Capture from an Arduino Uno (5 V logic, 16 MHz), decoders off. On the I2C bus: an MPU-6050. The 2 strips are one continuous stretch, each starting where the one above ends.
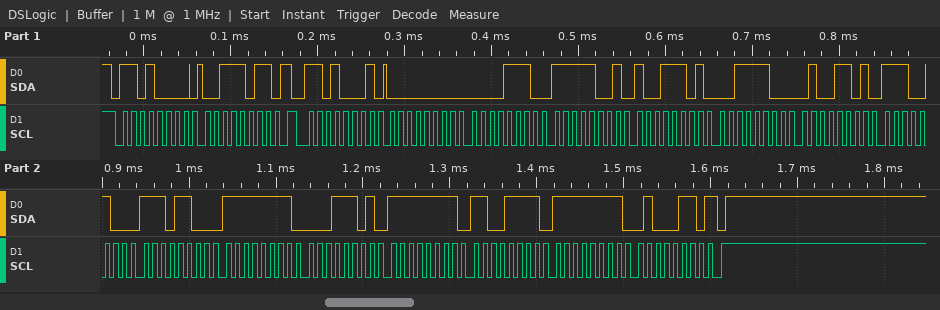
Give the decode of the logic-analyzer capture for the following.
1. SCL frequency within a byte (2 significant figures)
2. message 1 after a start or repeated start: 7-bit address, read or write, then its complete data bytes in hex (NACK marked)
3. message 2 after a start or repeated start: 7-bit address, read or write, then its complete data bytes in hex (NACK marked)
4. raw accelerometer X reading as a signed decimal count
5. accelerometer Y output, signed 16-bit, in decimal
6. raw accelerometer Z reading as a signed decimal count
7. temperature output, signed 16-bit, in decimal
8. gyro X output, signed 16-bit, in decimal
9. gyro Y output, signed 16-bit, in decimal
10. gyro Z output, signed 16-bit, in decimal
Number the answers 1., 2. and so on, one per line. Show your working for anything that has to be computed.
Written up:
1. 100 kHz
2. 0x68 write: 3B
3. 0x68 read: 00 0E F9 9D 3C 4D E4 EC FF 1D FF CF FF 46 NACK
4. 0x000E = 14
5. 0xF99D = -1635
6. 0x3C4D = 15437
7. 0xE4EC = -6932
8. 0xFF1D = -227
9. 0xFFCF = -49
10. 0xFF46 = -186
